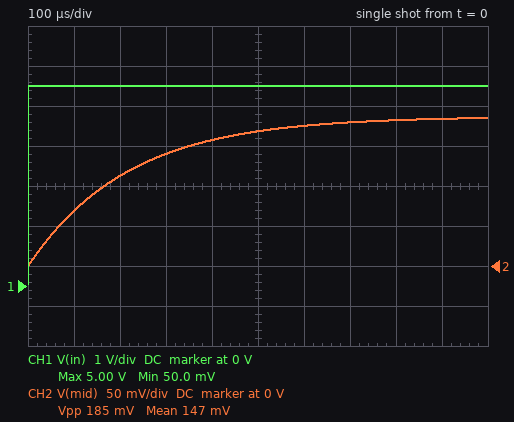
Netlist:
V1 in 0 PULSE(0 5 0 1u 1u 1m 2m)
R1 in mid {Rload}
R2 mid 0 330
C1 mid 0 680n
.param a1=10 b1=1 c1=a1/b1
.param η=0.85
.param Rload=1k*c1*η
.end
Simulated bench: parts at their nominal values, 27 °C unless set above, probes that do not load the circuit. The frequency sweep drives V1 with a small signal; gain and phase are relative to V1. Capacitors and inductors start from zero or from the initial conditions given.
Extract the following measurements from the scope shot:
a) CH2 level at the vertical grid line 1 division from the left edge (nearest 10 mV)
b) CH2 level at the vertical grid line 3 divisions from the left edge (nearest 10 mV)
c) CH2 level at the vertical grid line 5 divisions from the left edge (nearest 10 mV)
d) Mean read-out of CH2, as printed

70 mV
140 mV
170 mV
147 mV
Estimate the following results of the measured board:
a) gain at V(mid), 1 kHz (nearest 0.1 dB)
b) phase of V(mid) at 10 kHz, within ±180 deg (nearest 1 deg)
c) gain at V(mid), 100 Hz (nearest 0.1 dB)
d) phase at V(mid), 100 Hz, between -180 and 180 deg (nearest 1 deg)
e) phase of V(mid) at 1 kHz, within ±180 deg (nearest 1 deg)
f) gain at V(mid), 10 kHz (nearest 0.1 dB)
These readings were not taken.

-33.1 dB
-86 deg
-28.6 dB
-8 deg
-54 deg
-51.2 dB
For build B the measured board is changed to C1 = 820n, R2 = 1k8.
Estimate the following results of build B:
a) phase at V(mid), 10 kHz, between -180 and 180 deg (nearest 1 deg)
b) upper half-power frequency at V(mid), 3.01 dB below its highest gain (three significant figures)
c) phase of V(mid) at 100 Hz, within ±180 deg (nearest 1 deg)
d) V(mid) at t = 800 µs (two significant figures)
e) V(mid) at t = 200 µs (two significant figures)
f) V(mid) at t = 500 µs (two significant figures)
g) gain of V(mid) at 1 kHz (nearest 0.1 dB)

-89 deg
131 Hz
-37 deg
420 mV
130 mV
290 mV
-32.9 dB
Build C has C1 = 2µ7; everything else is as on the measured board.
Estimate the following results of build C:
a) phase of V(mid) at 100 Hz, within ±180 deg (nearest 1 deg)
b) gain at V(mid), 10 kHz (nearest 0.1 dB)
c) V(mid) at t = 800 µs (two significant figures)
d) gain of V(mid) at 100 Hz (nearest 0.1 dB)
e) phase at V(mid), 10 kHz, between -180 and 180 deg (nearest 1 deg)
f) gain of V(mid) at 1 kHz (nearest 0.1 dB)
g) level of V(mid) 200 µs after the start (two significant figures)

-28 deg
-63.2 dB
110 mV
-29.7 dB
-89 deg
-43.3 dB
39 mV
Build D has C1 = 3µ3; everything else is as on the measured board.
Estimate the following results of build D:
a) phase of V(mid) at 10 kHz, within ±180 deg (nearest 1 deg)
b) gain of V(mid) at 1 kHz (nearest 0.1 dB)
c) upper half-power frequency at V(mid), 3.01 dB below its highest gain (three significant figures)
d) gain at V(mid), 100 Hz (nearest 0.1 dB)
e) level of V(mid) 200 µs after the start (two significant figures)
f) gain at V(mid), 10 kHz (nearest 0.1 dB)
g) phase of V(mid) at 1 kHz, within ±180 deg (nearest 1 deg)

-89 deg
-45.0 dB
152 Hz
-30.1 dB
32 mV
-64.9 dB
-81 deg
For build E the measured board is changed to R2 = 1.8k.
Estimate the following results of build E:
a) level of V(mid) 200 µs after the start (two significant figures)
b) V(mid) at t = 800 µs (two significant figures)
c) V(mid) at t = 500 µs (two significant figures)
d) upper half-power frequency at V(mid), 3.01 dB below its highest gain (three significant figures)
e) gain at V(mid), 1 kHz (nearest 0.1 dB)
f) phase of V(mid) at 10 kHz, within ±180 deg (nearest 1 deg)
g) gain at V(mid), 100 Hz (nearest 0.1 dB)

160 mV
480 mV
340 mV
158 Hz
-31.3 dB
-89 deg
-16.6 dB
